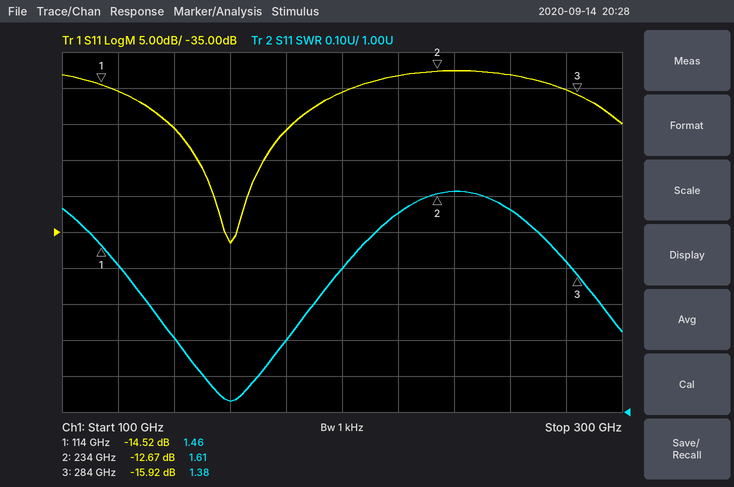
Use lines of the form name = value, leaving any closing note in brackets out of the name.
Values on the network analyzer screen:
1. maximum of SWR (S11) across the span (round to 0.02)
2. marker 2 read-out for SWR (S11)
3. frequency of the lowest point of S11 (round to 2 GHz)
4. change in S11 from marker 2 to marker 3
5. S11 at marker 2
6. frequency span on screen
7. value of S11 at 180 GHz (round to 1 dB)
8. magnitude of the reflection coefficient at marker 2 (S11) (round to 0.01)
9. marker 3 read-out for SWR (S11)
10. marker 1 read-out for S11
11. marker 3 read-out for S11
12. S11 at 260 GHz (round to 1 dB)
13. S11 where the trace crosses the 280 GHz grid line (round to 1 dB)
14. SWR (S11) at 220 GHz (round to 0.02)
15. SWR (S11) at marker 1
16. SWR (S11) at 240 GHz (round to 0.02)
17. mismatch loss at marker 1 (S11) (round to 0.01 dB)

maximum of SWR (S11) across the span = 1.62
marker 2 read-out for SWR = 1.61
frequency of the lowest point of S11 = 160 GHz
change in S11 from marker 2 to marker 3 = -3.25 dB
S11 at marker 2 = -12.67 dB
frequency span on screen = 200 GHz
value of S11 at 180 GHz = -21 dB
magnitude of the reflection coefficient at marker 2 (S11) = 0.23
marker 3 read-out for SWR = 1.38
marker 1 read-out for S11 = -14.52 dB
marker 3 read-out for S11 = -15.92 dB
S11 at 260 GHz = -13 dB
S11 where the trace crosses the 280 GHz grid line = -15 dB
SWR (S11) at 220 GHz = 1.56
SWR (S11) at marker 1 = 1.46
SWR (S11) at 240 GHz = 1.62
mismatch loss at marker 1 (S11) = 0.16 dB
